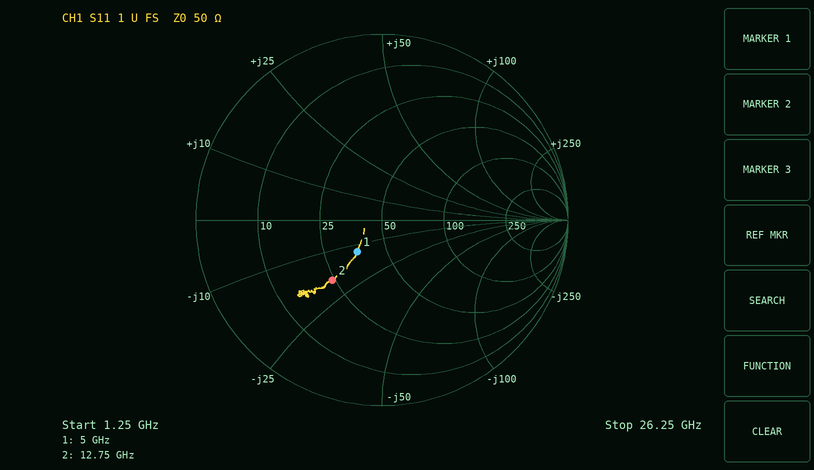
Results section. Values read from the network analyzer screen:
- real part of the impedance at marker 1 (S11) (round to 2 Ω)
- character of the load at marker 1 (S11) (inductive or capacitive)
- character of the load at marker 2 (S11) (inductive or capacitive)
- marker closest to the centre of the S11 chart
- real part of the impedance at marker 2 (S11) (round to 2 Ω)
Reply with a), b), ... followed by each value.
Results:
a) 36 Ω
b) capacitive
c) capacitive
d) marker 1
e) 24 Ω
